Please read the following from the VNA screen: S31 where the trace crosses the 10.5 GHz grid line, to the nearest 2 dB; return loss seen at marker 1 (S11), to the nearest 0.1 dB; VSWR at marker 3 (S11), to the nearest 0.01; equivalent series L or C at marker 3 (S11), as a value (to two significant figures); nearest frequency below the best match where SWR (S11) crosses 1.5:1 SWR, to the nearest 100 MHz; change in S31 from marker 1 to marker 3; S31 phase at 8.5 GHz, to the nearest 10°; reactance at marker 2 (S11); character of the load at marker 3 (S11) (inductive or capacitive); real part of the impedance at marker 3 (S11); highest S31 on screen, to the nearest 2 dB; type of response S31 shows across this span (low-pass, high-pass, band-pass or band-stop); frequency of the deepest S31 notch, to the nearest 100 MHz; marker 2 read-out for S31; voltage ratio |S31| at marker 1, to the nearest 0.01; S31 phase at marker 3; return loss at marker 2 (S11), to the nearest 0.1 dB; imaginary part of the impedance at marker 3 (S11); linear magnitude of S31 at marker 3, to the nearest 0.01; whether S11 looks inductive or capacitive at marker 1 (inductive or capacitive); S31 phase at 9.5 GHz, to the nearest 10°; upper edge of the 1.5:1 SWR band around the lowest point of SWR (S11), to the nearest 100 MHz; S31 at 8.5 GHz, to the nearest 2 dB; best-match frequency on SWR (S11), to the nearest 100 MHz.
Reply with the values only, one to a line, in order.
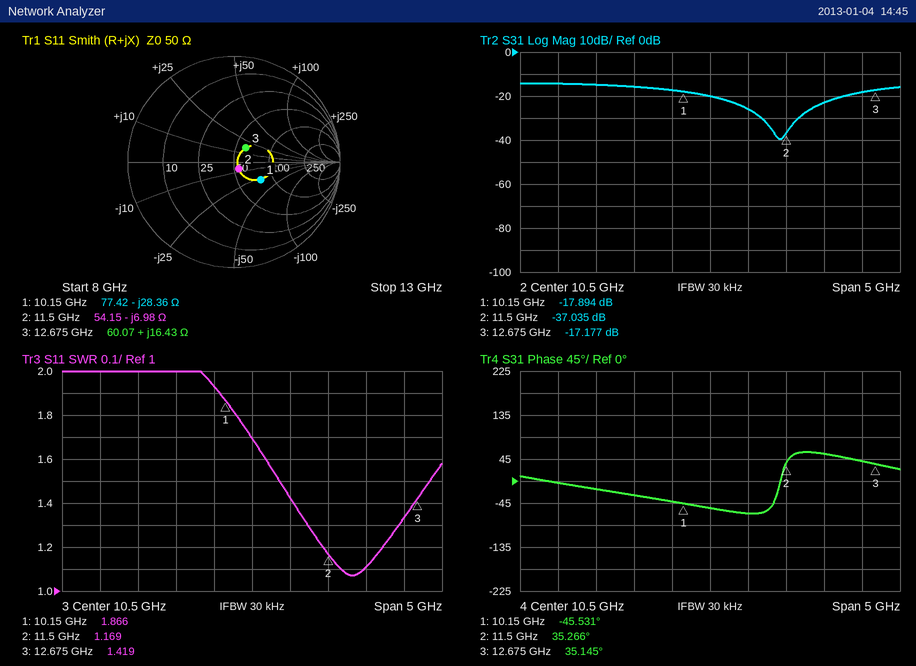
-20 dB
10.4 dB
1.42
210 pH
10.9 GHz
0.717 dB
0°
-6.98 Ω
inductive
60.07 Ω
-14 dB
band-stop
11.4 GHz
-37.035 dB
0.13
35.145°
22.2 dB
+16.43 Ω
0.14
capacitive
-30°
12.8 GHz
-14 dB
11.8 GHz
